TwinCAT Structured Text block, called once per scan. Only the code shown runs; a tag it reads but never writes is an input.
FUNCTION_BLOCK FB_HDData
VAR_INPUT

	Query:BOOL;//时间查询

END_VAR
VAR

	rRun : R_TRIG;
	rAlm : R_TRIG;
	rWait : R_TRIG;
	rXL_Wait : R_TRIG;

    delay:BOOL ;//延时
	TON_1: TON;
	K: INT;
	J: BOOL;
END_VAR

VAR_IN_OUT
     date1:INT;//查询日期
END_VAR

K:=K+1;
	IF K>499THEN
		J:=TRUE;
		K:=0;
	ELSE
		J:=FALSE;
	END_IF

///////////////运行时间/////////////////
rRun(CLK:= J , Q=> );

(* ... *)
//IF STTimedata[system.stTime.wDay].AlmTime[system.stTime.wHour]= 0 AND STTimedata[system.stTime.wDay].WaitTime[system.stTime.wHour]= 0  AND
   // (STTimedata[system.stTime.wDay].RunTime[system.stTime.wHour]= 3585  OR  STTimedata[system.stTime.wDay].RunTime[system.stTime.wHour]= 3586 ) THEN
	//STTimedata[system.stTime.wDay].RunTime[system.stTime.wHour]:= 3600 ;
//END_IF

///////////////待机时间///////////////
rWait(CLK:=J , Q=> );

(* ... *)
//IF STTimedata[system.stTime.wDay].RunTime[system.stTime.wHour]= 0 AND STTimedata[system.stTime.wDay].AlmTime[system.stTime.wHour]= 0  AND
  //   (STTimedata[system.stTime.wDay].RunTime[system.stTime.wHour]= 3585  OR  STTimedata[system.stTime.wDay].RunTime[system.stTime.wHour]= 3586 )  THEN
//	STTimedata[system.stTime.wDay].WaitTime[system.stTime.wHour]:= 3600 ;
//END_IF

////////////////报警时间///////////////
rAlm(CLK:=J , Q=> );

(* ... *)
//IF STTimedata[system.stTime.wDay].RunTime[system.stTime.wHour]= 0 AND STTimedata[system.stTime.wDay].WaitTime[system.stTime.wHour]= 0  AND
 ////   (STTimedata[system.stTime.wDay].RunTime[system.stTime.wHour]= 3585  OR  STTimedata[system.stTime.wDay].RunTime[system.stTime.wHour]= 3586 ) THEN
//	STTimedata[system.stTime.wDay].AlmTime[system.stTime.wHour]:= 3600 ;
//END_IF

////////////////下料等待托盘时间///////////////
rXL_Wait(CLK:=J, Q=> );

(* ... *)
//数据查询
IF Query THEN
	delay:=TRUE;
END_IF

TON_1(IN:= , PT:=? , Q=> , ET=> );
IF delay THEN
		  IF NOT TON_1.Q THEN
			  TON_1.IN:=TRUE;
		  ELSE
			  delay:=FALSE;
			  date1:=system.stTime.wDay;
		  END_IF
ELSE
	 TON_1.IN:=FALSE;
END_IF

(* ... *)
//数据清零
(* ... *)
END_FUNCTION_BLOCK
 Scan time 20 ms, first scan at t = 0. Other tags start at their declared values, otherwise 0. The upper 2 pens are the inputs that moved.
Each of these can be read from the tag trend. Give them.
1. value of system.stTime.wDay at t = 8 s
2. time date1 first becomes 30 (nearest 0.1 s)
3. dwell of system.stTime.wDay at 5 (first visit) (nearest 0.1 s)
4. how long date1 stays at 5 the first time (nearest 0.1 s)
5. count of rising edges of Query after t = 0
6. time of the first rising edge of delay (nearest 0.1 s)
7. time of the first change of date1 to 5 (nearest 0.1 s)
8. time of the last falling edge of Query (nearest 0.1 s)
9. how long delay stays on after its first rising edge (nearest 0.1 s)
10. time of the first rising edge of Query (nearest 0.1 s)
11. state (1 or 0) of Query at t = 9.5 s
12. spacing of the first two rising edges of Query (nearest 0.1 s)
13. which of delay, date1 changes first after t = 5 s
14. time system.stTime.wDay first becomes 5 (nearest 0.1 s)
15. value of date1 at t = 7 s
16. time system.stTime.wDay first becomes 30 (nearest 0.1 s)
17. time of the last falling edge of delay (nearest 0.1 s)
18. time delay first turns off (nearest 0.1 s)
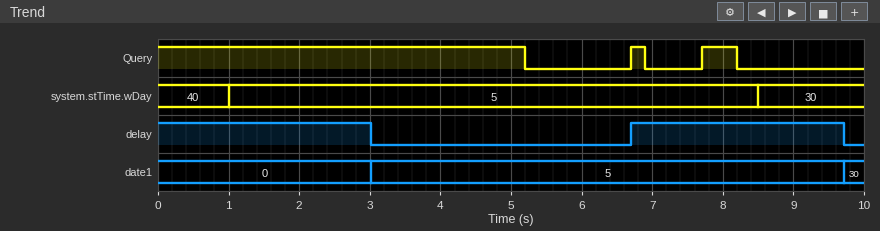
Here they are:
5
9.7 s
7.5 s
6.7 s
2
6.7 s
3.0 s
8.2 s
3.0 s
6.7 s
0
1.0 s
delay
1.0 s
5
8.5 s
9.7 s
3.0 s
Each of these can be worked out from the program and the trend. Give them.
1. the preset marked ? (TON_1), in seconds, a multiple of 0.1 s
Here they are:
3.0 s
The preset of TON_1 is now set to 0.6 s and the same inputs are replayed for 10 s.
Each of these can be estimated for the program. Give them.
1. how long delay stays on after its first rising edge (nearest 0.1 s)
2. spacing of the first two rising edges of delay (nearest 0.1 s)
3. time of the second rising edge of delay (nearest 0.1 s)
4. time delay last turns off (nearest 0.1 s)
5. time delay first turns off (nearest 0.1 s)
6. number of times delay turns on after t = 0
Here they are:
0.6 s
1.0 s
7.7 s
8.3 s
0.6 s
2
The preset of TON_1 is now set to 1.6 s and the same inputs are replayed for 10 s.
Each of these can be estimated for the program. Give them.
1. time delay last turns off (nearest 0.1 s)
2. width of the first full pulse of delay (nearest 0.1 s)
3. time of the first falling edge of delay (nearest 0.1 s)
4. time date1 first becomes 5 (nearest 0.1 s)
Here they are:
8.3 s
1.6 s
1.6 s
1.6 s
